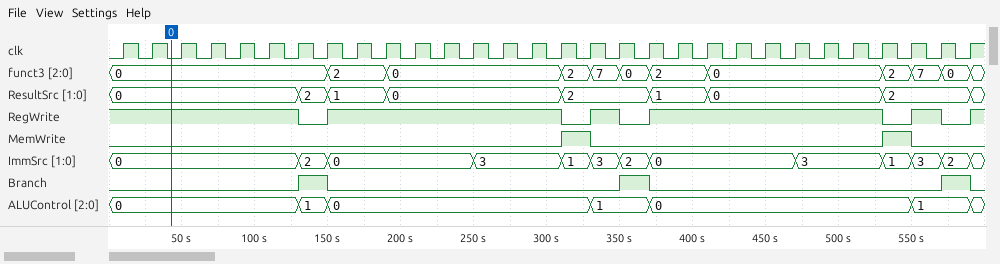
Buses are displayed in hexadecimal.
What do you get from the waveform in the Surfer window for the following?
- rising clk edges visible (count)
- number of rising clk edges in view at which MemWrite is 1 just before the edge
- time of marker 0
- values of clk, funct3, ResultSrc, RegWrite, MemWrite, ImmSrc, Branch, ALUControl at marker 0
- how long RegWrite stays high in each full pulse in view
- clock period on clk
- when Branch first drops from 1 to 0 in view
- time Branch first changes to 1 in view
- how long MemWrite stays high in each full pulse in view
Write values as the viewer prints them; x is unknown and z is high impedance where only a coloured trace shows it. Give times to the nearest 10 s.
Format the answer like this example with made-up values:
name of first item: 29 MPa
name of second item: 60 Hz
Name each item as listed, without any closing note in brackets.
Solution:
rising clk edges visible: 30
number of rising clk edges in view at which MemWrite is 1 just before the edge: 2
time of marker 0: 40 s
values of clk, funct3, ResultSrc, RegWrite, MemWrite, ImmSrc, Branch, ALUControl at marker 0: clk=0, funct3=0, ResultSrc=0, RegWrite=1, MemWrite=0, ImmSrc=0, Branch=0, ALUControl=0
how long RegWrite stays high in each full pulse in view: 160 s, 20 s, 160 s, 20 s
clock period on clk: 20 s
when Branch first drops from 1 to 0 in view: 150 s
time Branch first changes to 1 in view: 130 s
how long MemWrite stays high in each full pulse in view: 20 s, 20 s
